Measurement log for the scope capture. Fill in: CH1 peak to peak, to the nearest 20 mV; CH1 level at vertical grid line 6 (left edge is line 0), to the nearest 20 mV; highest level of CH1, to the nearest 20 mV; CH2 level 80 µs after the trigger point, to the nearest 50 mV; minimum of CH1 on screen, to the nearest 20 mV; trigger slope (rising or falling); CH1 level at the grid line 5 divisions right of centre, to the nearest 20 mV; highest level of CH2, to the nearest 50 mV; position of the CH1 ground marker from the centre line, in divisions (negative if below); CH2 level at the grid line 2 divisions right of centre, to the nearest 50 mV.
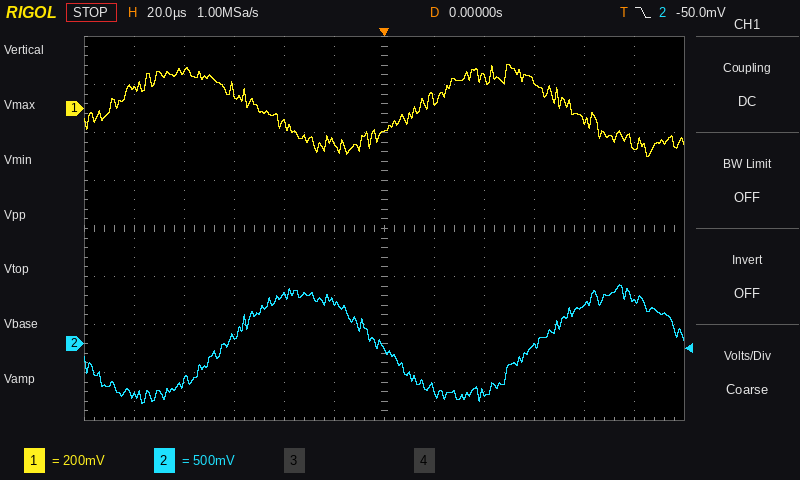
380 mV
-100 mV
180 mV
400 mV
-200 mV
falling
-160 mV
600 mV
+2.5 div
-500 mV
